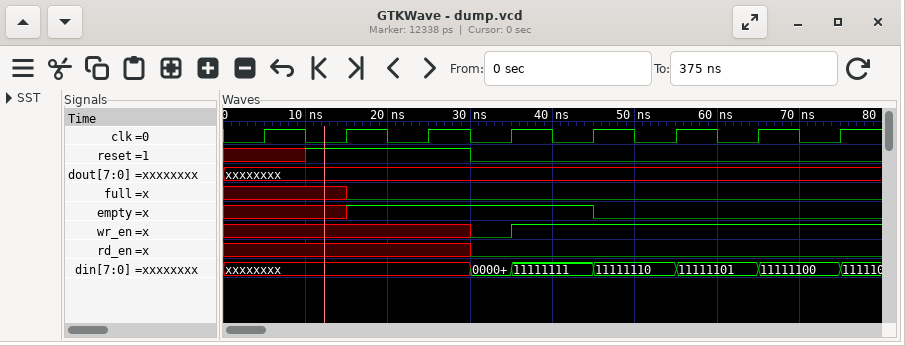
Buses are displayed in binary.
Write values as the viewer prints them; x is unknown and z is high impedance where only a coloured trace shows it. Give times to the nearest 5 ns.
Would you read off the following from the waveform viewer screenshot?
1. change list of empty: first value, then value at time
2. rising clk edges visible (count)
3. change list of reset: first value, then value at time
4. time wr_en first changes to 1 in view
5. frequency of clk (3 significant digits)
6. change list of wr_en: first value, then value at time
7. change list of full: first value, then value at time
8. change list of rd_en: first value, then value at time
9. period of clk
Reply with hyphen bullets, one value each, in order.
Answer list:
- x, 1 at 15 ns, 0 at 45 ns
- 8
- x, 1 at 10 ns, 0 at 30 ns
- 35 ns
- 100 MHz
- x, 0 at 30 ns, 1 at 35 ns
- x, 0 at 15 ns
- x, 0 at 30 ns
- 10 ns
